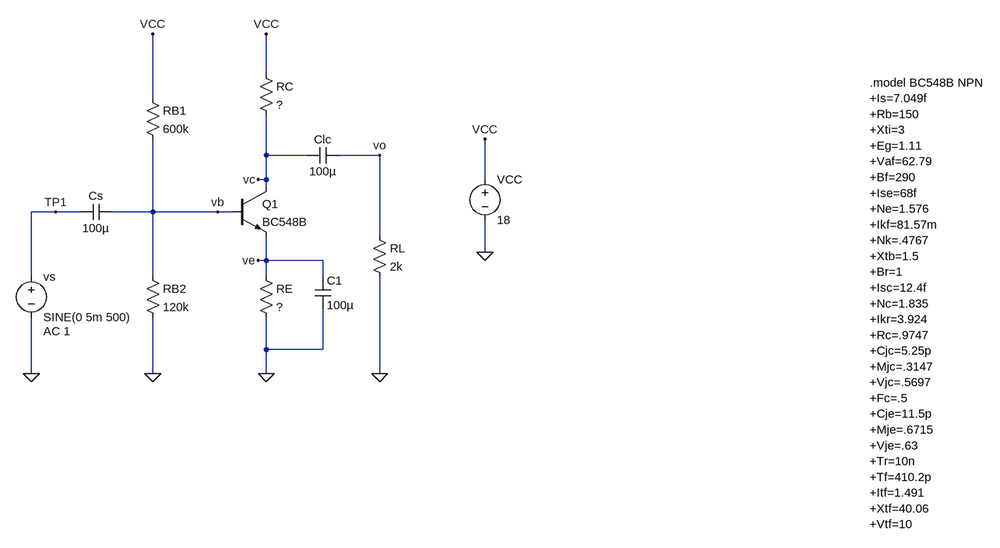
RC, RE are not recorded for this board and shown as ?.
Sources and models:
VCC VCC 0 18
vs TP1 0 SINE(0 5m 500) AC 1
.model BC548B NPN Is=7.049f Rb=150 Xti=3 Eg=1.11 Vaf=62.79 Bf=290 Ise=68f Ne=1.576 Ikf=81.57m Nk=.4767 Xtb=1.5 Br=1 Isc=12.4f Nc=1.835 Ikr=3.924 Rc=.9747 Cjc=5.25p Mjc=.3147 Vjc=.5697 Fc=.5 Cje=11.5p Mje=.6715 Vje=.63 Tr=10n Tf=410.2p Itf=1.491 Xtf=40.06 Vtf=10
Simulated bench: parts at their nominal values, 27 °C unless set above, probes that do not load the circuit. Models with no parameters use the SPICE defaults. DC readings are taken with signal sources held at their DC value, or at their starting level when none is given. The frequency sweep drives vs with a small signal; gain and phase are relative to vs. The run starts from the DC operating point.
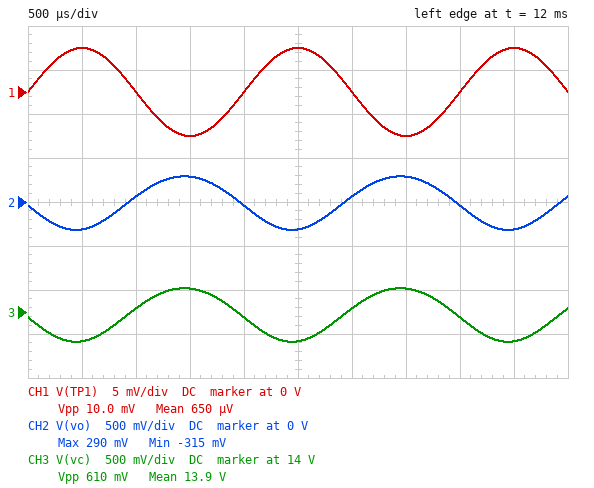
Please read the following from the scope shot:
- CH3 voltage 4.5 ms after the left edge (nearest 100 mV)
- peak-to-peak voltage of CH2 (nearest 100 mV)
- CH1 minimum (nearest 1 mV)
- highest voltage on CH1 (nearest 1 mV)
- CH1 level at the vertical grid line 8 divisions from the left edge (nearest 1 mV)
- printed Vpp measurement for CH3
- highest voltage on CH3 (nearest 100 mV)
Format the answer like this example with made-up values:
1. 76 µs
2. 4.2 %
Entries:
1. 13.7 V
2. 600 mV
3. -5 mV
4. 5 mV
5. 0 V
6. 610 mV
7. 14.3 V
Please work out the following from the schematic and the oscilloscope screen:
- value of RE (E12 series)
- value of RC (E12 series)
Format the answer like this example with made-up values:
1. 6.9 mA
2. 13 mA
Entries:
1. 1.2 kΩ
2. 2.7 kΩ
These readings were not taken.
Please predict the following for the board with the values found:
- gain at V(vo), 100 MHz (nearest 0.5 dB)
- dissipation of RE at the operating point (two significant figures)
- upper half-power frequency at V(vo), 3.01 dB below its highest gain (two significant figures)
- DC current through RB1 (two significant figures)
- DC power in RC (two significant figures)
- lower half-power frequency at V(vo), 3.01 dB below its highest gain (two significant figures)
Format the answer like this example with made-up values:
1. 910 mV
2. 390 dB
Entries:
1. 10.0 dB
2. 2.7 mW
3. 5.6 MHz
4. 26 µA
5. 6.0 mW
6. 88 Hz
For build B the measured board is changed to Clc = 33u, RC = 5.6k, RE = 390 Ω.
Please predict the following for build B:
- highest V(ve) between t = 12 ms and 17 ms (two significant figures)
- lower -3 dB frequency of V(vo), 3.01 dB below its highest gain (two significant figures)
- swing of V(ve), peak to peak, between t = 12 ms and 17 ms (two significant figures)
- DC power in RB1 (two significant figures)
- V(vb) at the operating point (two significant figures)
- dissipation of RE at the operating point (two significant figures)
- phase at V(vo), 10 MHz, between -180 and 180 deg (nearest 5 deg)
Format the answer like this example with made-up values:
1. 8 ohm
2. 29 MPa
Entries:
1. 1.1 V
2. 160 Hz
3. 2.8 mV
4. 440 µW
5. 1.8 V
6. 3.2 mW
7. 95 deg
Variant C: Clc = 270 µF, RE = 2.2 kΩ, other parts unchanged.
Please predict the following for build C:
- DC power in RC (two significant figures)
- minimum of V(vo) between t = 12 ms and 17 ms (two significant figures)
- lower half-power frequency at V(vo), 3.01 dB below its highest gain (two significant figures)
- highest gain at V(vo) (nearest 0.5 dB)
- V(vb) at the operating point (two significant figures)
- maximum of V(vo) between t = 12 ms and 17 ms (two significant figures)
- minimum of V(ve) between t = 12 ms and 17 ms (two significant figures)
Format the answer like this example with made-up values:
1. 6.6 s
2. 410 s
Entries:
1. 2.2 mW
2. -200 mV
3. 55 Hz
4. 32.0 dB
5. 2.7 V
6. 180 mV
7. 2.0 V
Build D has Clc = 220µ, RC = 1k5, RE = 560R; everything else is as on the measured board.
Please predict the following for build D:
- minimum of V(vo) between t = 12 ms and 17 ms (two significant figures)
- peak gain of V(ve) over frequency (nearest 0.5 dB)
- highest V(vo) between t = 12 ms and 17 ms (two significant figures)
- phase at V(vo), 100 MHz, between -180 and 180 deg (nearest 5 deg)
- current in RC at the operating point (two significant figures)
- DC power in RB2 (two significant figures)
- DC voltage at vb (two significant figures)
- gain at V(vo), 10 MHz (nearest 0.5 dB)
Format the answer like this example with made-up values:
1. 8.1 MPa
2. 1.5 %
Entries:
1. -380 mV
2. 0 dB
3. 350 mV
4. 75 deg
5. 2.5 mA
6. 37 µW
7. 2.1 V
8. 30.0 dB
